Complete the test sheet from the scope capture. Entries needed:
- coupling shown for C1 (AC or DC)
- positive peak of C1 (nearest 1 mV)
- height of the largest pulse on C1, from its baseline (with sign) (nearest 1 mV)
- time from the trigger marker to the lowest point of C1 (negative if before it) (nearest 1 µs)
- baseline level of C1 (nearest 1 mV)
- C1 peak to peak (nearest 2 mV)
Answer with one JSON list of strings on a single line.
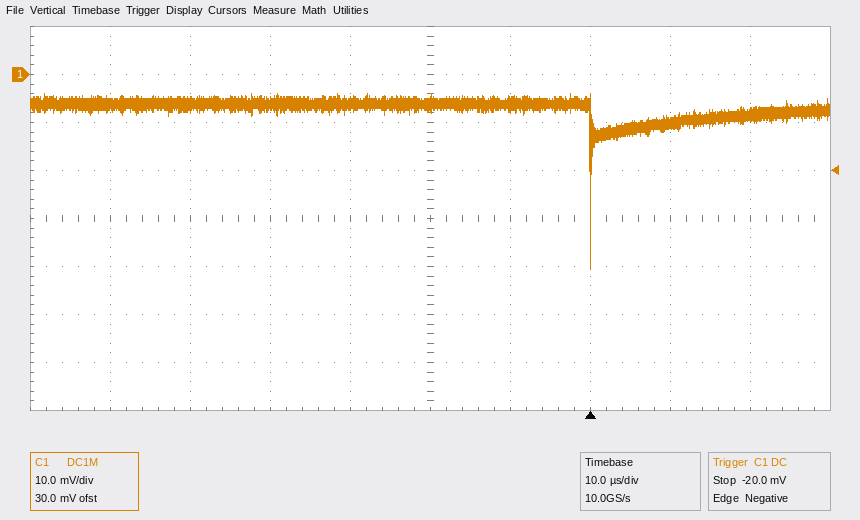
["DC", "-4 mV", "-34 mV", "0 µs", "-6 mV", "36 mV"]
